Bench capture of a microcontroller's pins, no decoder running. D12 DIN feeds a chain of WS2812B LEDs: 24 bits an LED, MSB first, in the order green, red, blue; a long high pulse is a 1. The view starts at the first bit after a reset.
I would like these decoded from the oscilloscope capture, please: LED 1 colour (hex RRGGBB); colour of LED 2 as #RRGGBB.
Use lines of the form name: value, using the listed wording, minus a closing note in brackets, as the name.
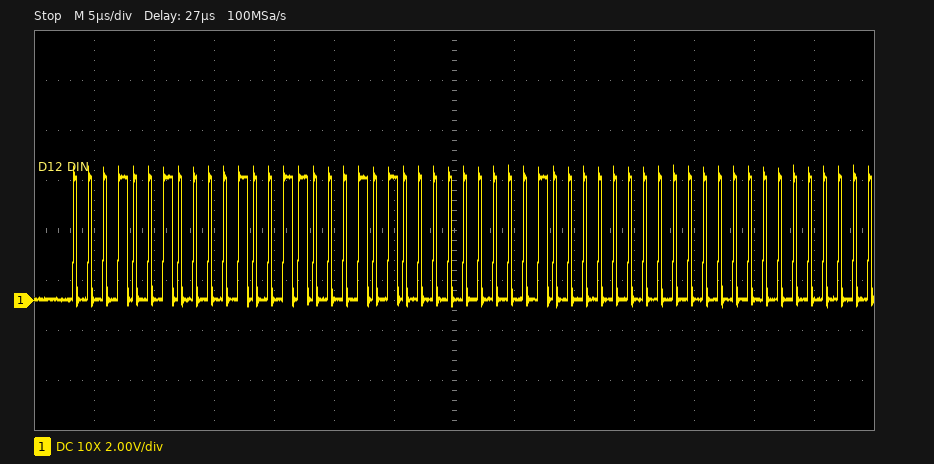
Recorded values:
LED 1 colour: #131214
colour of LED 2 as #RRGGBB: #000100
